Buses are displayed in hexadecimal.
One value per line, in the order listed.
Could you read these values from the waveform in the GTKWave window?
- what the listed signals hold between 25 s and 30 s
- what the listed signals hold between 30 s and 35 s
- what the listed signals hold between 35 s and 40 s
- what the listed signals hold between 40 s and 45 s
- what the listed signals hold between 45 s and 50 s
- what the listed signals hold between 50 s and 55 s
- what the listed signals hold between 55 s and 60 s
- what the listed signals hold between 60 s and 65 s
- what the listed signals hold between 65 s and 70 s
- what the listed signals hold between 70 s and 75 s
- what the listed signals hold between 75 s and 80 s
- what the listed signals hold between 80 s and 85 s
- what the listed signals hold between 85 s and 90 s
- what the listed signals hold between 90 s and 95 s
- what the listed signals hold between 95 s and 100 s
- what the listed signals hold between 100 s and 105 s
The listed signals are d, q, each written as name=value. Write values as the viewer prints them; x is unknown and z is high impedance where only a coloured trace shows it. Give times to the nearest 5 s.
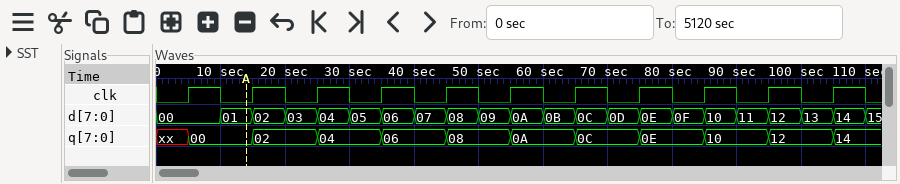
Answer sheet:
d=04, q=04
d=05, q=04
d=06, q=06
d=07, q=06
d=08, q=08
d=09, q=08
d=0A, q=0A
d=0B, q=0A
d=0C, q=0C
d=0D, q=0C
d=0E, q=0E
d=0F, q=0E
d=10, q=10
d=11, q=10
d=12, q=12
d=13, q=12
